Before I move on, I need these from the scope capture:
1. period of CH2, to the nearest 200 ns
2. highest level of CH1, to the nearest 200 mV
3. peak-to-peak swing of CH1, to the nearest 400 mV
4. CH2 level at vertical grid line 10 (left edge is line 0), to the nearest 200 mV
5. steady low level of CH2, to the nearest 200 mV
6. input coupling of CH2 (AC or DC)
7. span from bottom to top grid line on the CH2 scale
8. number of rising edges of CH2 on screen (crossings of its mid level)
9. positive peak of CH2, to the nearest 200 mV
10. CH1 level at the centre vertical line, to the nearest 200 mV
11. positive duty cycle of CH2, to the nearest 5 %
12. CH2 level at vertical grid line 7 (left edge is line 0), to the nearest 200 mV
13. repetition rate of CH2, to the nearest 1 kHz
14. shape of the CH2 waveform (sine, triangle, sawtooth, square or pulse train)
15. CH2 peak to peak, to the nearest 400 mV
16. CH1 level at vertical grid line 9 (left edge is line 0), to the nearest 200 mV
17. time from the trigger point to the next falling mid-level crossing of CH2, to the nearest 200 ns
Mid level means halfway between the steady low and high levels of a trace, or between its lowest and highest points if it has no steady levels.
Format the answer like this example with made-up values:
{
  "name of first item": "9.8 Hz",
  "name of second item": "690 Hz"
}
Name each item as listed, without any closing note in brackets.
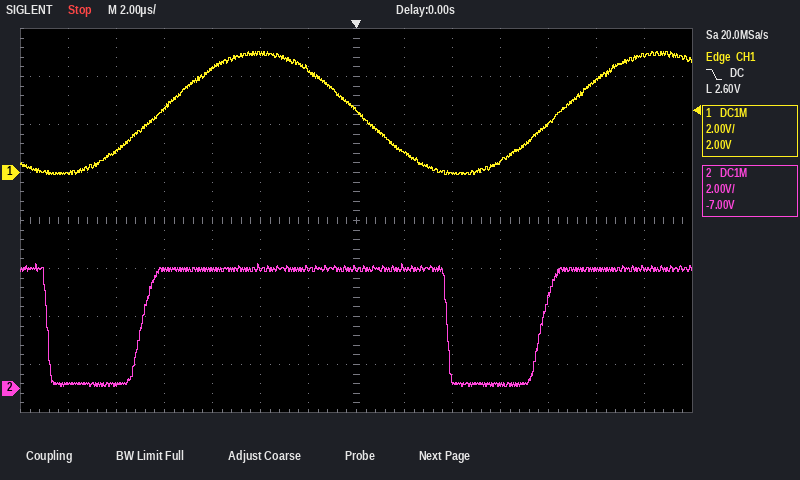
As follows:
{
  "period of CH2, to the nearest 200 ns": "16.6 µs",
  "highest level of CH1, to the nearest 200 mV": "5.0 V",
  "peak-to-peak swing of CH1, to the nearest 400 mV": "5.2 V",
  "CH2 level at vertical grid line 10 (left edge is line 0), to the nearest 200 mV": "200 mV",
  "steady low level of CH2, to the nearest 200 mV": "200 mV",
  "input coupling of CH2": "DC",
  "span from bottom to top grid line on the CH2 scale": "16 V",
  "number of rising edges of CH2 on screen": "2",
  "positive peak of CH2, to the nearest 200 mV": "5.2 V",
  "CH1 level at the centre vertical line, to the nearest 200 mV": "2.6 V",
  "positive duty cycle of CH2, to the nearest 5 %": "75 %",
  "CH2 level at vertical grid line 7 (left edge is line 0), to the nearest 200 mV": "5.0 V",
  "repetition rate of CH2, to the nearest 1 kHz": "60 kHz",
  "shape of the CH2 waveform": "pulse train",
  "CH2 peak to peak, to the nearest 400 mV": "5.2 V",
  "CH1 level at vertical grid line 9 (left edge is line 0), to the nearest 200 mV": "0.0 V",
  "time from the trigger point to the next falling mid-level crossing of CH2, to the nearest 200 ns": "3.8 µs"
}
